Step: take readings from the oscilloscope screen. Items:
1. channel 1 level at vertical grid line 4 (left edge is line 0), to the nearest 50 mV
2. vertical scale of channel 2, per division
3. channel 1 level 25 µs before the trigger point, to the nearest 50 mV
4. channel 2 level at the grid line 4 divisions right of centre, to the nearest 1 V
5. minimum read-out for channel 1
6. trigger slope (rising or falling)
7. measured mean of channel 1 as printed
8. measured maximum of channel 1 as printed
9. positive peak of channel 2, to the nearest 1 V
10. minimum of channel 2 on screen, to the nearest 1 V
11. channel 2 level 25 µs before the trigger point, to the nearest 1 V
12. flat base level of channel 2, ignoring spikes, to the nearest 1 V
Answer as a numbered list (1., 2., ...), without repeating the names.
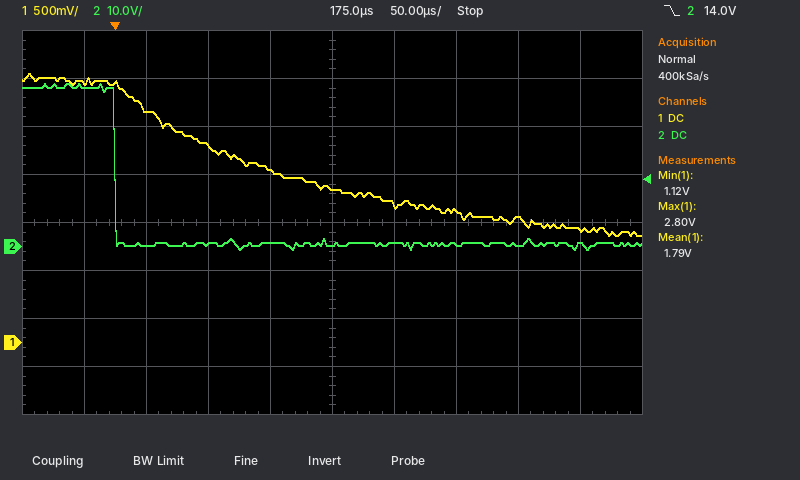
1. 1.80 V
2. 10 V
3. 2.70 V
4. 1 V
5. 1.12 V
6. falling
7. 1.79 V
8. 2.80 V
9. 34 V
10. -1 V
11. 33 V
12. 1 V
